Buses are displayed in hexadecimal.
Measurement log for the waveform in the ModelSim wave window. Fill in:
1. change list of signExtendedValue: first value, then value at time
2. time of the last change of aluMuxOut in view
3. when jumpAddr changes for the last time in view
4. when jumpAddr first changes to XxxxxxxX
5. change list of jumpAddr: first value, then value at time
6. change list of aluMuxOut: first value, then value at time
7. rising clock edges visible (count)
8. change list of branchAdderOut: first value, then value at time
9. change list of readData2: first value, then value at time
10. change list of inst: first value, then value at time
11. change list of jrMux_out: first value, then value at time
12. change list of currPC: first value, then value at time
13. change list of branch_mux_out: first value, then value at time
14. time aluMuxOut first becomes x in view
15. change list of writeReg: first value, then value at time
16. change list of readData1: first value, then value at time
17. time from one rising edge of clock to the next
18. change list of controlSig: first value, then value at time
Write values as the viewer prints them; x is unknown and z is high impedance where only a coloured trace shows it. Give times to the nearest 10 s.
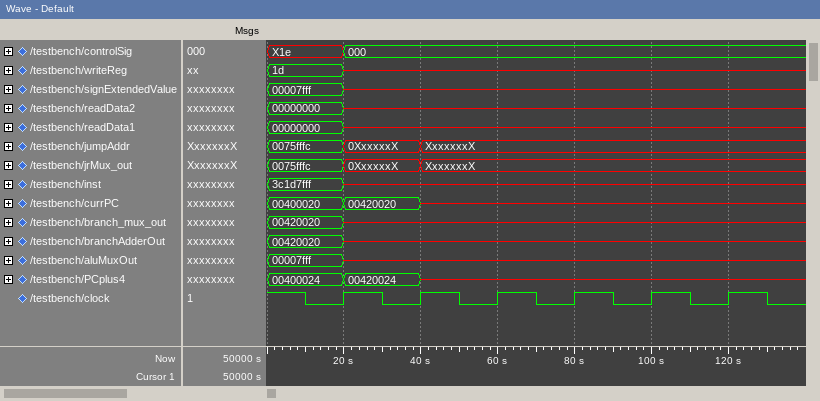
00007fff, x at 20 s
20 s
40 s
40 s
0075fffc, 0XxxxxxX at 20 s, XxxxxxxX at 40 s
00007fff, x at 20 s
6
00420020, x at 20 s
00000000, x at 20 s
3c1d7fff, x at 20 s
0075fffc, 0XxxxxxX at 20 s, XxxxxxxX at 40 s
00400020, 00420020 at 20 s, x at 40 s
00420020, x at 20 s
20 s
1d, x at 20 s
00000000, x at 20 s
20 s
X1e, 000 at 20 s
